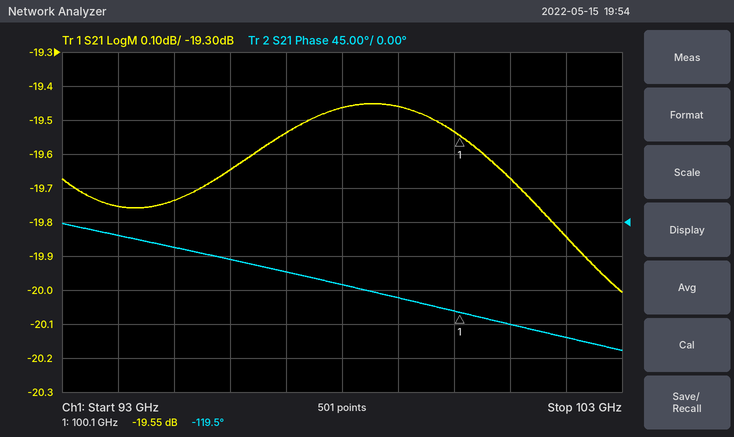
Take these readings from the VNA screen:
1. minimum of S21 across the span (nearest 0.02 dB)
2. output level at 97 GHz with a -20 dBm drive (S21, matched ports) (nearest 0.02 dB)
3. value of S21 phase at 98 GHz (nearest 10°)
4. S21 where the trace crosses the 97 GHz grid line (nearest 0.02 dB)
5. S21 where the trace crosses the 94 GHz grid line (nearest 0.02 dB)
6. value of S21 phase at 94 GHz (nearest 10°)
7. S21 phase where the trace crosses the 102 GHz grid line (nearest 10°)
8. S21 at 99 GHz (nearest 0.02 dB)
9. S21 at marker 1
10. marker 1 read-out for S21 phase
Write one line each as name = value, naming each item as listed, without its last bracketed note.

minimum of S21 across the span = -20.00 dB
output level at 97 GHz with a -20 dBm drive (S21, matched ports) = -39.54 dBm
value of S21 phase at 98 GHz = -80°
S21 where the trace crosses the 97 GHz grid line = -19.54 dB
S21 where the trace crosses the 94 GHz grid line = -19.76 dB
value of S21 phase at 94 GHz = -20°
S21 phase where the trace crosses the 102 GHz grid line = -150°
S21 at 99 GHz = -19.46 dB
S21 at marker 1 = -19.55 dB
marker 1 read-out for S21 phase = -119.5°
